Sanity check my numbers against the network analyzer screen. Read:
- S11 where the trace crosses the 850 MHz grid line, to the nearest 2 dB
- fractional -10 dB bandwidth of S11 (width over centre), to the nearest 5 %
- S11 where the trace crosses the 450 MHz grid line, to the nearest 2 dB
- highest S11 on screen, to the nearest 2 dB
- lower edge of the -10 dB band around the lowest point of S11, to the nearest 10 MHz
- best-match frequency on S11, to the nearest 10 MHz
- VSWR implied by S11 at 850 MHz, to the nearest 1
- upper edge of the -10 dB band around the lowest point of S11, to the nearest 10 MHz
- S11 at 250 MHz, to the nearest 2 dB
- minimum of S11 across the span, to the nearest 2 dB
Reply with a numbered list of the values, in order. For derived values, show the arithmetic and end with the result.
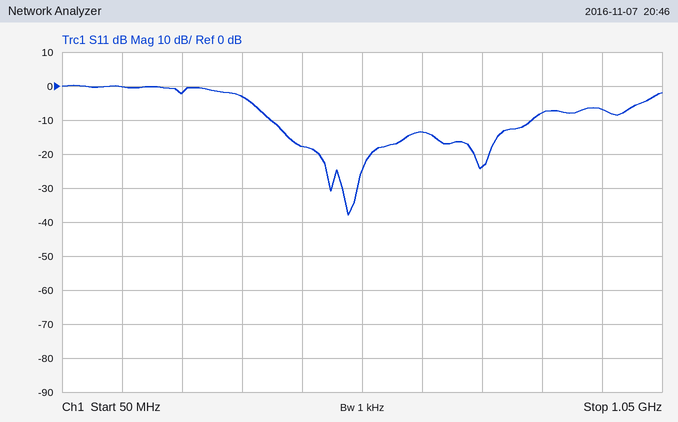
1. -8 dB
2. 430 MHz / 615 MHz ≈ 70 %
3. -18 dB
4. 0 dB
5. 400 MHz
6. 530 MHz
7. |Γ| = 10^(-8/20) = 0.3981; VSWR = (1 + 0.3981)/(1 − 0.3981) ≈ 2
8. 830 MHz
9. -2 dB
10. -38 dB
